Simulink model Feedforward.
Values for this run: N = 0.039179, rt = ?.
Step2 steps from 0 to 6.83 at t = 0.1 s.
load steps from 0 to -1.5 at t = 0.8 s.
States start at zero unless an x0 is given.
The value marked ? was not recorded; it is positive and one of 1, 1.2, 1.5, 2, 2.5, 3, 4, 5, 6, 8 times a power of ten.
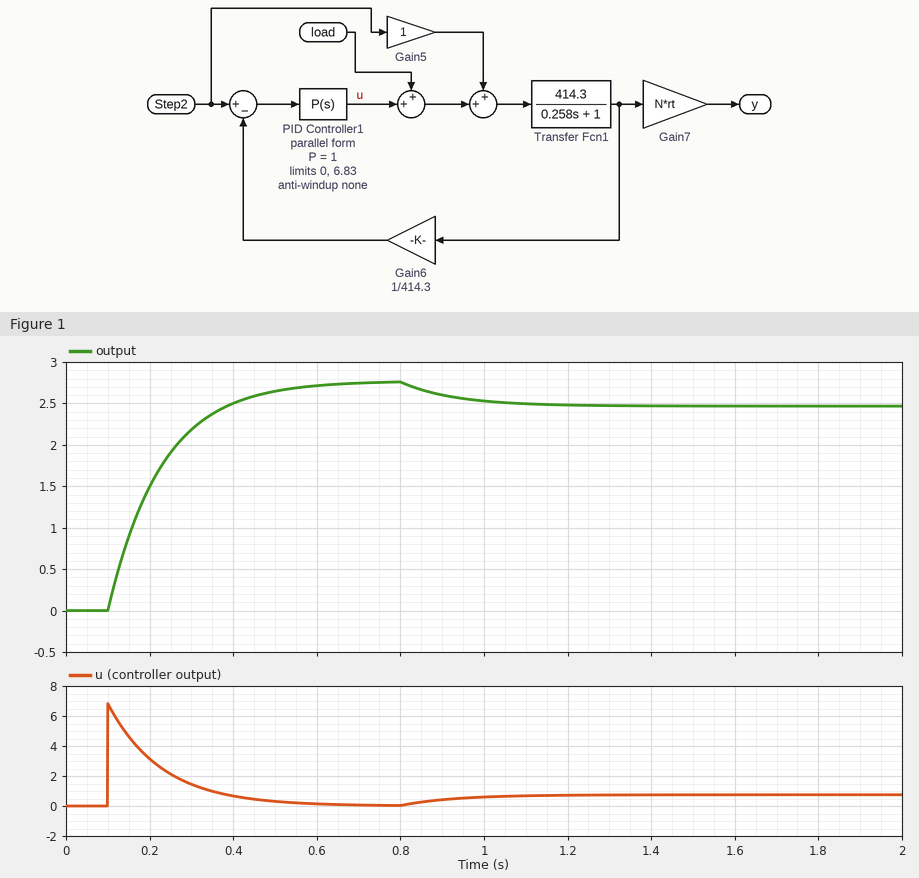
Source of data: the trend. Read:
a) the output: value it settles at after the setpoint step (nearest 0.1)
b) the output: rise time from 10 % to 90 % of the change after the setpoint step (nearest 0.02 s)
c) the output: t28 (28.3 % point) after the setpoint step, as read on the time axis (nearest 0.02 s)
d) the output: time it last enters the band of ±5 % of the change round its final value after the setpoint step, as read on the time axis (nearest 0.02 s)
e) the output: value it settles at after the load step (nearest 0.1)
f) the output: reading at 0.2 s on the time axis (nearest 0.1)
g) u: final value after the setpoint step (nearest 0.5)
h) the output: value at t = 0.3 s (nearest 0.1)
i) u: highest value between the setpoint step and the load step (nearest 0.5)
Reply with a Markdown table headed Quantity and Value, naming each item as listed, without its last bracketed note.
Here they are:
| Quantity | Value |
|---|---|
| the output: value it settles at after the setpoint step | 2.8 |
| the output: rise time from 10 % to 90 % of the change after the setpoint step | 0.28 s |
| the output: t28 (28.3 % point) after the setpoint step, as read on the time axis | 0.14 s |
| the output: time it last enters the band of ±5 % of the change round its final value after the setpoint step, as read on the time axis | 0.48 s |
| the output: value it settles at after the load step | 2.5 |
| the output: reading at 0.2 s on the time axis | 1.5 |
| u: final value after the setpoint step | 0.0 |
| the output: value at t = 0.3 s | 2.2 |
| u: highest value between the setpoint step and the load step | 7.0 |
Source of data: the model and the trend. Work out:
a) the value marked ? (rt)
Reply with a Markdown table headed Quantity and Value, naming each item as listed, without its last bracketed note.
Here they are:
| Quantity | Value |
|---|---|
| the value marked ? | 0.025 |
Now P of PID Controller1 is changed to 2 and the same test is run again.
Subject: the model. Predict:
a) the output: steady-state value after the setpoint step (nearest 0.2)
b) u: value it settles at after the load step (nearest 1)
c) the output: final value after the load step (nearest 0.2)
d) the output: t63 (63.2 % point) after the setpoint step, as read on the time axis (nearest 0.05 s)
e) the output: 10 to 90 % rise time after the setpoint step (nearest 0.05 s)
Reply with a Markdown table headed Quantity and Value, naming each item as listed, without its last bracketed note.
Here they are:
| Quantity | Value |
|---|---|
| the output: steady-state value after the setpoint step | 2.8 |
| u: value it settles at after the load step | 1 |
| the output: final value after the load step | 2.6 |
| the output: t63 (63.2 % point) after the setpoint step, as read on the time axis | 0.20 s |
| the output: 10 to 90 % rise time after the setpoint step | 0.20 s |
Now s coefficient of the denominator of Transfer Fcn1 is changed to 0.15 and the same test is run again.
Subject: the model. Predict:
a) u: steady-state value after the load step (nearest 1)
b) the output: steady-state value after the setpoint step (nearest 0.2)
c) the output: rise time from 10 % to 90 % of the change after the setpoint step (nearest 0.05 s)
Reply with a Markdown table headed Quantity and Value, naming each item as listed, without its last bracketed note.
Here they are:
| Quantity | Value |
|---|---|
| u: steady-state value after the load step | 1 |
| the output: steady-state value after the setpoint step | 2.8 |
| the output: rise time from 10 % to 90 % of the change after the setpoint step | 0.15 s |
